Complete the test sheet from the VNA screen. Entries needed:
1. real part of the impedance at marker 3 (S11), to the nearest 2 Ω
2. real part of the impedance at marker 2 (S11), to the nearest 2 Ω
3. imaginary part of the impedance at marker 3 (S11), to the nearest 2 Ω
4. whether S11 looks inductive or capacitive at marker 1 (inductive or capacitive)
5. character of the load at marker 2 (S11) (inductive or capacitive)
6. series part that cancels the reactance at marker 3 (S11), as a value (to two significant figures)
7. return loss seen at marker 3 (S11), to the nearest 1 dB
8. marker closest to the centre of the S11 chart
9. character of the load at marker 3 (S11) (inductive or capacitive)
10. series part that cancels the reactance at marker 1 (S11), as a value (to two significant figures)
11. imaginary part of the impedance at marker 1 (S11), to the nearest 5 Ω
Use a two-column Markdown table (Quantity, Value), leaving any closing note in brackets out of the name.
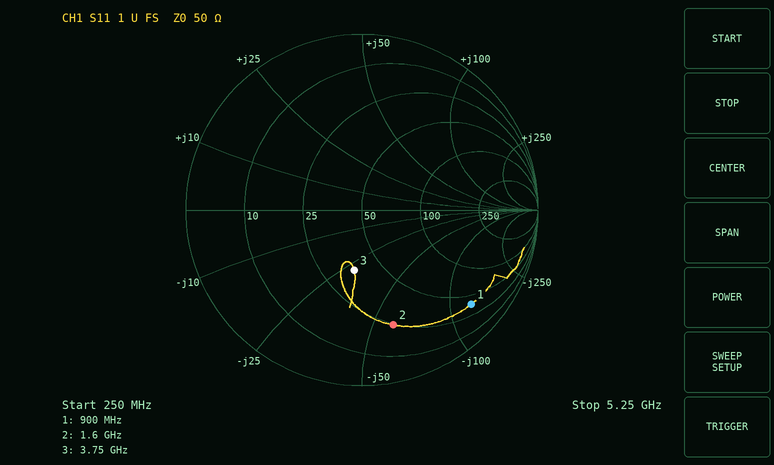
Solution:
| Quantity | Value |
|---|---|
| real part of the impedance at marker 3 (S11), to the nearest 2 Ω | 36 Ω |
| real part of the impedance at marker 2 (S11), to the nearest 2 Ω | 24 Ω |
| imaginary part of the impedance at marker 3 (S11), to the nearest 2 Ω | -28 Ω |
| whether S11 looks inductive or capacitive at marker 1 | capacitive |
| character of the load at marker 2 (S11) | capacitive |
| series part that cancels the reactance at marker 3 (S11), as a value | 1.2 nH |
| return loss seen at marker 3 (S11), to the nearest 1 dB | 9 dB |
| marker closest to the centre of the S11 chart | marker 3 |
| character of the load at marker 3 (S11) | capacitive |
| series part that cancels the reactance at marker 1 (S11), as a value | 22 nH |
| imaginary part of the impedance at marker 1 (S11), to the nearest 5 Ω | -125 Ω |
